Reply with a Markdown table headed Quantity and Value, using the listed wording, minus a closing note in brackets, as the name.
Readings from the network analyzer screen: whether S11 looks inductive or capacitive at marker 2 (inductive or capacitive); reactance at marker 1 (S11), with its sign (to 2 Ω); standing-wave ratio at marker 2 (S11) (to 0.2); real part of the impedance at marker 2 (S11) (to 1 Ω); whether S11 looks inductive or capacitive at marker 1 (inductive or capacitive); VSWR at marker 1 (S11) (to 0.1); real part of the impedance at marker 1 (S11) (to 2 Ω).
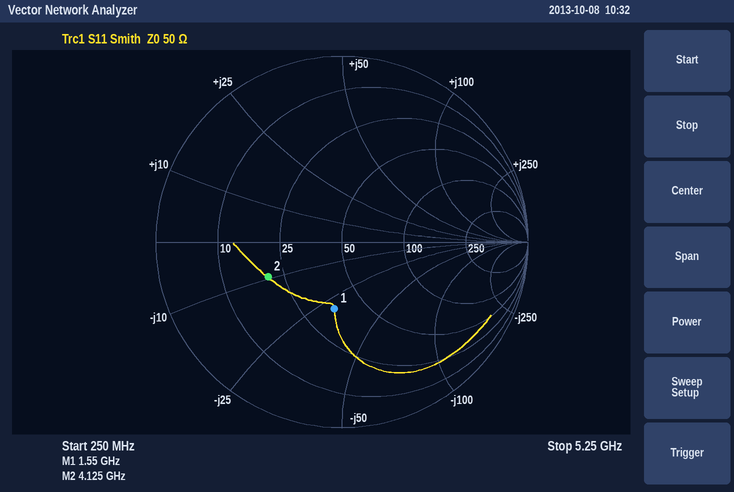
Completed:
| Quantity | Value |
|---|---|
| whether S11 looks inductive or capacitive at marker 2 | capacitive |
| reactance at marker 1 (S11), with its sign | -30 Ω |
| standing-wave ratio at marker 2 (S11) | 2.6 |
| real part of the impedance at marker 2 (S11) | 20 Ω |
| whether S11 looks inductive or capacitive at marker 1 | capacitive |
| VSWR at marker 1 (S11) | 2.1 |
| real part of the impedance at marker 1 (S11) | 36 Ω |
